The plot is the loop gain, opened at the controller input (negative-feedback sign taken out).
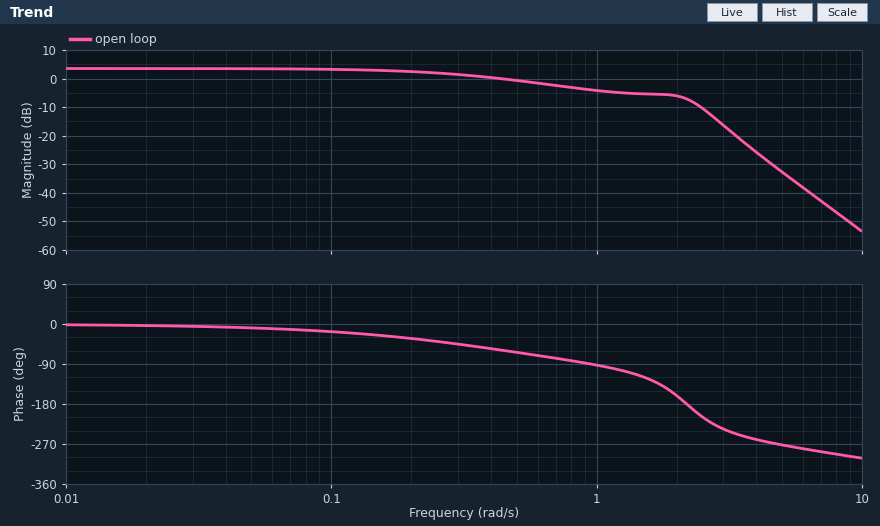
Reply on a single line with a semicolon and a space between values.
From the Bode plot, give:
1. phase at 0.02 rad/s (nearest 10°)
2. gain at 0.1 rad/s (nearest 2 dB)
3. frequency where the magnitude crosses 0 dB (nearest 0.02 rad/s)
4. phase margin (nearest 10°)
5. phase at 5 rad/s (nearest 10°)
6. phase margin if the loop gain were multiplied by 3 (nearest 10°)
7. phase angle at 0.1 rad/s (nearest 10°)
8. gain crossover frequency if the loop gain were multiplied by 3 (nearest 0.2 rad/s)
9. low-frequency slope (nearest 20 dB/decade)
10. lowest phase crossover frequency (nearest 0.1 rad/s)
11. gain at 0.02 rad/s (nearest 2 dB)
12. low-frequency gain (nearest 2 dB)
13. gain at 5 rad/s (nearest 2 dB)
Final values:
0°; 4 dB; 0.44 rad/s; 120°; -270°; -20°; -20°; 2.4 rad/s; 0 dB/decade; 2.2 rad/s; 4 dB; 4 dB; -32 dB
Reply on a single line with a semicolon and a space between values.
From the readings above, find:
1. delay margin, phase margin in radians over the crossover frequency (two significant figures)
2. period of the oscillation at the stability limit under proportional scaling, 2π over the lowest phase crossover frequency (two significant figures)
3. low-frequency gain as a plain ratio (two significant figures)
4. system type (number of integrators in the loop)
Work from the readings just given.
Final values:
4.8 s; 2.9 s; 1.6; 0
